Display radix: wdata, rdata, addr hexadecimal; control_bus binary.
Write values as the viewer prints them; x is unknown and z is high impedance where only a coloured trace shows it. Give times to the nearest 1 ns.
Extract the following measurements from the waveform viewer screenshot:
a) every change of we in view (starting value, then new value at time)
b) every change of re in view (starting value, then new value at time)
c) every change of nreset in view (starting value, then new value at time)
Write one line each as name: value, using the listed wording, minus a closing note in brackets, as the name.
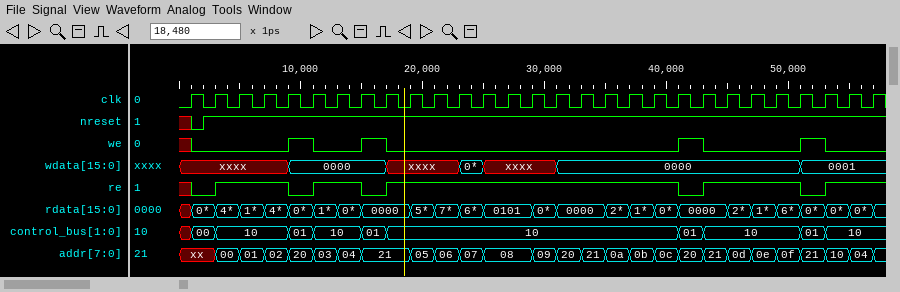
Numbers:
every change of we in view: x, 0 at 1 ns, 1 at 9 ns, 0 at 11 ns, 1 at 15 ns, 0 at 17 ns, 1 at 41 ns, 0 at 43 ns, 1 at 51 ns, 0 at 53 ns
every change of re in view: x, 0 at 1 ns, 1 at 3 ns, 0 at 9 ns, 1 at 11 ns, 0 at 15 ns, 1 at 17 ns, 0 at 41 ns, 1 at 43 ns, 0 at 51 ns, 1 at 53 ns
every change of nreset in view: x, 0 at 1 ns, 1 at 2 ns
